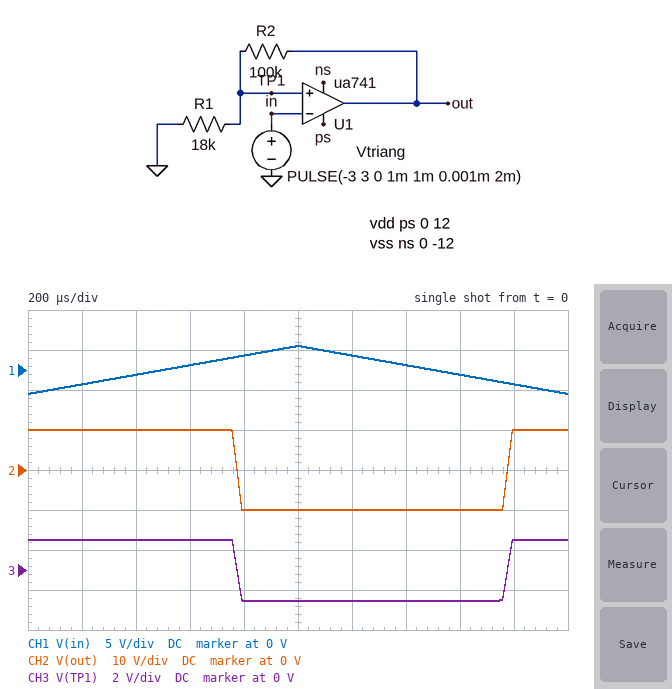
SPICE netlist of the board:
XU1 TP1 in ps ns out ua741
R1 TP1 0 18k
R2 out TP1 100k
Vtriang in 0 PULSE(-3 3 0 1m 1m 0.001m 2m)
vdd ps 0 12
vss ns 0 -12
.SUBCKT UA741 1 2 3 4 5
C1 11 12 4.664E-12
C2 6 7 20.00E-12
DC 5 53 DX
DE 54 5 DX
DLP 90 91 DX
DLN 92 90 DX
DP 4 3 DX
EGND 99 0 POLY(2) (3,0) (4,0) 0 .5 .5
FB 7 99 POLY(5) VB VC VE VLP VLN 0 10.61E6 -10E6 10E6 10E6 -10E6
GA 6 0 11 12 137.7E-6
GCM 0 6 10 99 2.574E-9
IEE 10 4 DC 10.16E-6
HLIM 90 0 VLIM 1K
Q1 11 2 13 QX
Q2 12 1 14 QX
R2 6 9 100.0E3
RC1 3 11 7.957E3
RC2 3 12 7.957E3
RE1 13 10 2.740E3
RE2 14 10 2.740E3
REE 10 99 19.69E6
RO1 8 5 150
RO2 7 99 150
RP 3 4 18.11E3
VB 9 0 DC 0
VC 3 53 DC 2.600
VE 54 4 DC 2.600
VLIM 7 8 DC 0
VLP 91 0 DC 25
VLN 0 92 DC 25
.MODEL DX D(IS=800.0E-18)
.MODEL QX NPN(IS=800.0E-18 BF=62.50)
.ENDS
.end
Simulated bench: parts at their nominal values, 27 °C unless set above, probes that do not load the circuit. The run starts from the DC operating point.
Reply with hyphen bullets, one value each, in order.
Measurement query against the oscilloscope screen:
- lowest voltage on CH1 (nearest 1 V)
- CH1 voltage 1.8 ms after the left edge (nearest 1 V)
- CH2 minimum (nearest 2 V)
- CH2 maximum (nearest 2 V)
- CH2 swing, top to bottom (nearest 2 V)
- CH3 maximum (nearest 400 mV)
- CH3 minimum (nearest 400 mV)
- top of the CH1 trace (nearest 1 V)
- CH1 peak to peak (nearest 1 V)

- -3 V
- -2 V
- -10 V
- 10 V
- 20 V
- 1.6 V
- -1.6 V
- 3 V
- 6 V
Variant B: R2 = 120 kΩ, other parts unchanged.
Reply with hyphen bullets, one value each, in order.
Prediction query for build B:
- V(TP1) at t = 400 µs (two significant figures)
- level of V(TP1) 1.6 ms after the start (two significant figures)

- 1.3 V
- -1.3 V
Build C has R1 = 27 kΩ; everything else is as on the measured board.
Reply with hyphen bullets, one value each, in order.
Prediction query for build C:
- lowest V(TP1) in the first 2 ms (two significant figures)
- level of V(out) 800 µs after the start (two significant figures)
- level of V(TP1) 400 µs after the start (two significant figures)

- -2.1 V
- 10 V
- 2.1 V
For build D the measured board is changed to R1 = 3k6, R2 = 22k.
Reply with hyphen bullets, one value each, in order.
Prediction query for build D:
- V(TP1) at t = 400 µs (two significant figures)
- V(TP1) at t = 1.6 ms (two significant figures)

- 1.4 V
- -1.4 V
